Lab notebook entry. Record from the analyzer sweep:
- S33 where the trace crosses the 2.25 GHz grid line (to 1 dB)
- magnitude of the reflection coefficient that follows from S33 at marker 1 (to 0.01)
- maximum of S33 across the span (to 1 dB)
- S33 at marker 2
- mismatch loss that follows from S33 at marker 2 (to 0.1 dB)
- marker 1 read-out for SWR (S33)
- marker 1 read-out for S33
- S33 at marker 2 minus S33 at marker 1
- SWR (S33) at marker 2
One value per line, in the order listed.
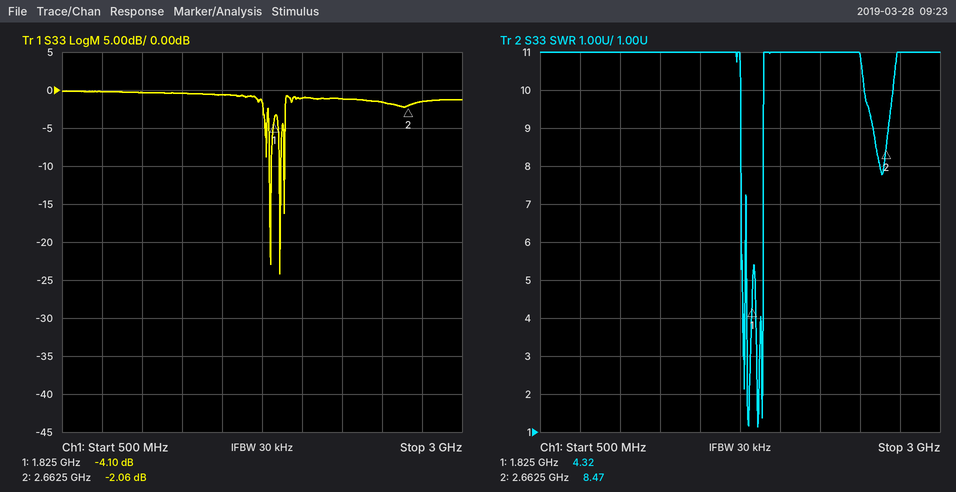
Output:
-1 dB
0.62
0 dB
-2.06 dB
4.2 dB
4.32
-4.10 dB
2.04 dB
8.47
